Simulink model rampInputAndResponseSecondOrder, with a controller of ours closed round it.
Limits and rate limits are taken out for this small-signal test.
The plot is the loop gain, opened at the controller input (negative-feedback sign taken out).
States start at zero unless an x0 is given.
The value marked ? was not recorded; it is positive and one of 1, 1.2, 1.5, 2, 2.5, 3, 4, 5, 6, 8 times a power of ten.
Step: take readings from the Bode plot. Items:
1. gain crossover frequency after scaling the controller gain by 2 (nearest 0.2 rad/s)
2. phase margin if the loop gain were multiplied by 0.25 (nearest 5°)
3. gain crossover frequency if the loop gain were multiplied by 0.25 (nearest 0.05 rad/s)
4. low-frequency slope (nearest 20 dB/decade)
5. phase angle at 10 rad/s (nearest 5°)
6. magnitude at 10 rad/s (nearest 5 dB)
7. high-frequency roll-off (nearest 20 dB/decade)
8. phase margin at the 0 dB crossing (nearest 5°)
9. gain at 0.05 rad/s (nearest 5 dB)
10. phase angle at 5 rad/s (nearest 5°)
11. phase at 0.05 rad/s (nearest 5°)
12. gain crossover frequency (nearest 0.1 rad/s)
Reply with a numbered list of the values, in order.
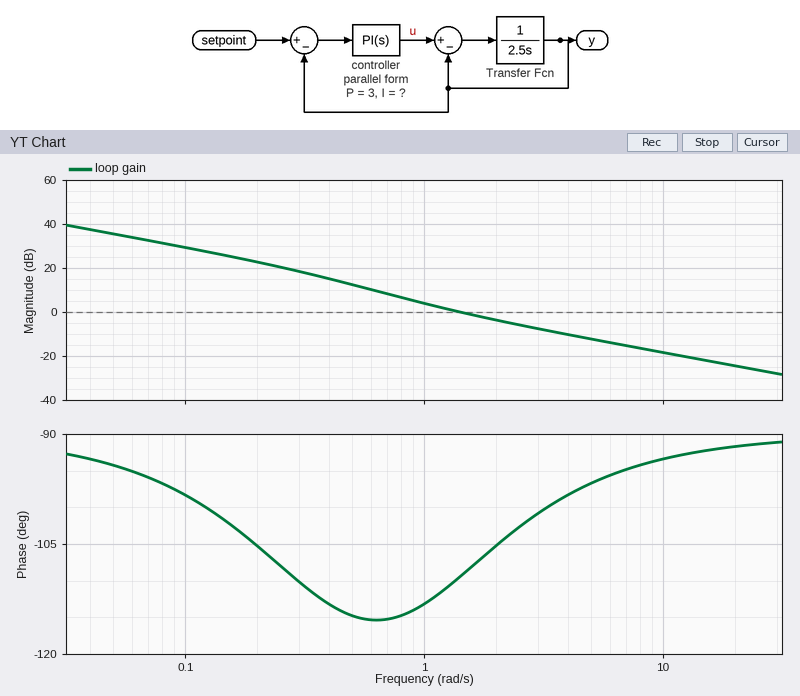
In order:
1. 2.6 rad/s
2. 65°
3. 0.50 rad/s
4. -20 dB/decade
5. -95°
6. -20 dB
7. -20 dB/decade
8. 70°
9. 35 dB
10. -95°
11. -95°
12. 1.4 rad/s
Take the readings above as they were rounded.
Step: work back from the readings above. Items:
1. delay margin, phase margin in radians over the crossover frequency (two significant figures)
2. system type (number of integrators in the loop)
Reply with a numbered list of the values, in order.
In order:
1. 0.87 s
2. 1
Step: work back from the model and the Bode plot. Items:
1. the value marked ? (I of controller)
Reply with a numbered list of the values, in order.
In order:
1. 3
